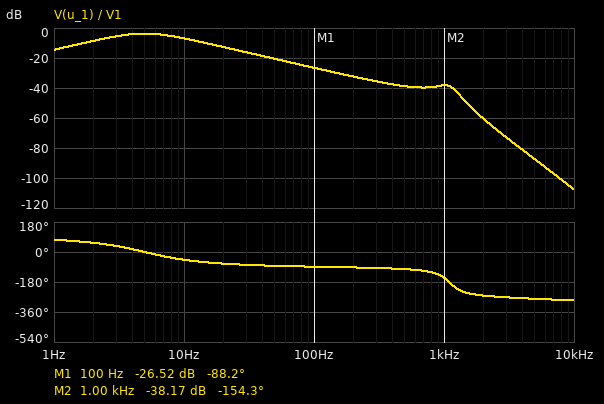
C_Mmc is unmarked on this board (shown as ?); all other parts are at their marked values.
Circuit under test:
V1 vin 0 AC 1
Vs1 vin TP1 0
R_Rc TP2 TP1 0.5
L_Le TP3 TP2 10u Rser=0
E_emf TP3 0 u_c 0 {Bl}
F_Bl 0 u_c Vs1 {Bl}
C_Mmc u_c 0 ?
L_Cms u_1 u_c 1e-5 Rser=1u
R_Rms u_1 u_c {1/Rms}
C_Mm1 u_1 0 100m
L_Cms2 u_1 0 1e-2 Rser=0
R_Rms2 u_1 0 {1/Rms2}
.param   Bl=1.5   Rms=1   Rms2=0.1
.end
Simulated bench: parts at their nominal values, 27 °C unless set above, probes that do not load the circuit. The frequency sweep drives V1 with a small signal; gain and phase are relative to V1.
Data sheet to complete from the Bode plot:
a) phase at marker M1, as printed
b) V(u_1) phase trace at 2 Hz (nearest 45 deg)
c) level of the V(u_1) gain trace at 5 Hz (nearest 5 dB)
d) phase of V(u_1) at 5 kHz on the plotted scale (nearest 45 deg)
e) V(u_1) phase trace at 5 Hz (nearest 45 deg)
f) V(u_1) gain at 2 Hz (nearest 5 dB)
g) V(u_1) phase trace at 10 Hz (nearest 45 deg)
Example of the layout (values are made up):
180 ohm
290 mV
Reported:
-88.2 deg
45 deg
-5 dB
-270 deg
0 deg
-10 dB
-45 deg
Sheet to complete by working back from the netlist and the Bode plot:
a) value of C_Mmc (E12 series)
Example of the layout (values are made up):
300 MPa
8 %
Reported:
2.2 mF
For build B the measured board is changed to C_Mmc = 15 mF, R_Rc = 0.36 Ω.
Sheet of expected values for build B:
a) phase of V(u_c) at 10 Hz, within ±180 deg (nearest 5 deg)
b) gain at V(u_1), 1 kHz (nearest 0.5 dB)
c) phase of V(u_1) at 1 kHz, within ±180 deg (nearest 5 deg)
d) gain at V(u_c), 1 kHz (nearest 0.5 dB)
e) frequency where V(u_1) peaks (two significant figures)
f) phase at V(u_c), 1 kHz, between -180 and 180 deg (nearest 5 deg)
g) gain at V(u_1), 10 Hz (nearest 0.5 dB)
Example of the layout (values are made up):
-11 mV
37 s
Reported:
-40 deg
-57.0 dB
90 deg
-25.5 dB
4.7 Hz
-95 deg
-6.0 dB
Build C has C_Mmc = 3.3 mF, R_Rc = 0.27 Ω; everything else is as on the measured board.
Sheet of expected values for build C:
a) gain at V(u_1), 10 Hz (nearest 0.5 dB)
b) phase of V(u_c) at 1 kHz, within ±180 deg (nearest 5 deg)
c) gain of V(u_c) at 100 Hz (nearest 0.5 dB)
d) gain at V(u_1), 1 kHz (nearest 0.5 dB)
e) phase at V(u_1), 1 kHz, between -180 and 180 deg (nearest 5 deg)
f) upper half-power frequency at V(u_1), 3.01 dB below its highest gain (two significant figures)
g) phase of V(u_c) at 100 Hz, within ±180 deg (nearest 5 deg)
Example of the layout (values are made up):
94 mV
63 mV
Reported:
-5.0 dB
-30 deg
-25.5 dB
-36.5 dB
155 deg
15 Hz
-85 deg
